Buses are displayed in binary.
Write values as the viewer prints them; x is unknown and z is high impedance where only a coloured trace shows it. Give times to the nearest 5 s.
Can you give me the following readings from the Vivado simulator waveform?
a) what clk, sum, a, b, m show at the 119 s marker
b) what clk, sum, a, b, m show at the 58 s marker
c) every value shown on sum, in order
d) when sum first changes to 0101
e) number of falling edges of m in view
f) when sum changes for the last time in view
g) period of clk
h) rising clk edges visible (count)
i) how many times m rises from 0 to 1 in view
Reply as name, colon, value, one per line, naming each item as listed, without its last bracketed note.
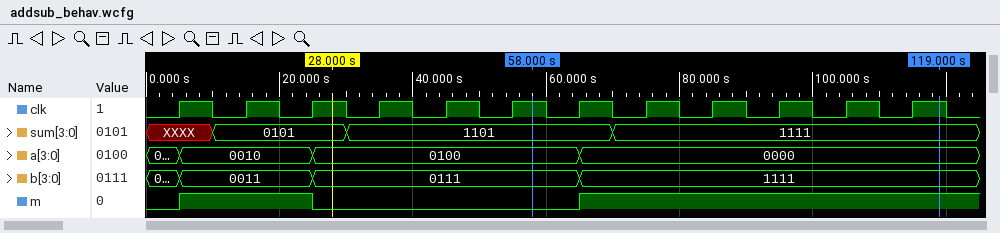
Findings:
what clk, sum, a, b, m show at the 119 s marker: clk=1, sum=1111, a=0000, b=1111, m=1
what clk, sum, a, b, m show at the 58 s marker: clk=1, sum=1101, a=0100, b=0111, m=0
every value shown on sum, in order: XXXX, 0101, 1101, 1111
when sum first changes to 0101: 10 s
number of falling edges of m in view: 1
when sum changes for the last time in view: 70 s
period of clk: 10 s
rising clk edges visible: 12
how many times m rises from 0 to 1 in view: 2
